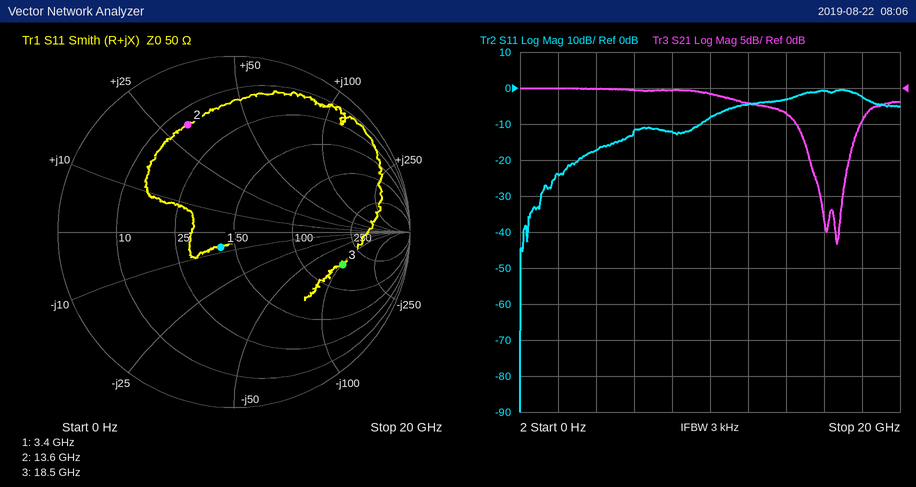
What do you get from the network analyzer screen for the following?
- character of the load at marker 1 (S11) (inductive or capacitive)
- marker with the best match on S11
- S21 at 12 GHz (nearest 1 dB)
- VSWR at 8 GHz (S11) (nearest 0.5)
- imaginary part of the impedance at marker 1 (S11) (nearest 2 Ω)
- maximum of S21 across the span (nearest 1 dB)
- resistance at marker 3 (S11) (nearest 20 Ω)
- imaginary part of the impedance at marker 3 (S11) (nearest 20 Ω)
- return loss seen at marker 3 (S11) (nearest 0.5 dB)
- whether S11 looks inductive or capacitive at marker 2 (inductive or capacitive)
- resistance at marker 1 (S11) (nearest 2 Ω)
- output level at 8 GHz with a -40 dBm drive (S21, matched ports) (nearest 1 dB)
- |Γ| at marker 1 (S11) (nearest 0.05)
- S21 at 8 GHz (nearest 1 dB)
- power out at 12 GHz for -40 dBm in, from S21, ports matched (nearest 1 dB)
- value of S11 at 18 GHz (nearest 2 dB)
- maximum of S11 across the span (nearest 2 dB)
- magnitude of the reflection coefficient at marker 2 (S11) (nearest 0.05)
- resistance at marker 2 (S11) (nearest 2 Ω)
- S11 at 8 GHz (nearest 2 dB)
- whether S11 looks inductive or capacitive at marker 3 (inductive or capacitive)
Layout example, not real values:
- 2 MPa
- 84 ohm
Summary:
- capacitive
- marker 1
- -2 dB
- 1.5
- -8 Ω
- 0 dB
- 160 Ω
- -100 Ω
- 4.0 dB
- inductive
- 42 Ω
- -40 dBm
- 0.10
- 0 dB
- -42 dBm
- -2 dB
- 0 dB
- 0.65
- 14 Ω
- -12 dB
- capacitive
